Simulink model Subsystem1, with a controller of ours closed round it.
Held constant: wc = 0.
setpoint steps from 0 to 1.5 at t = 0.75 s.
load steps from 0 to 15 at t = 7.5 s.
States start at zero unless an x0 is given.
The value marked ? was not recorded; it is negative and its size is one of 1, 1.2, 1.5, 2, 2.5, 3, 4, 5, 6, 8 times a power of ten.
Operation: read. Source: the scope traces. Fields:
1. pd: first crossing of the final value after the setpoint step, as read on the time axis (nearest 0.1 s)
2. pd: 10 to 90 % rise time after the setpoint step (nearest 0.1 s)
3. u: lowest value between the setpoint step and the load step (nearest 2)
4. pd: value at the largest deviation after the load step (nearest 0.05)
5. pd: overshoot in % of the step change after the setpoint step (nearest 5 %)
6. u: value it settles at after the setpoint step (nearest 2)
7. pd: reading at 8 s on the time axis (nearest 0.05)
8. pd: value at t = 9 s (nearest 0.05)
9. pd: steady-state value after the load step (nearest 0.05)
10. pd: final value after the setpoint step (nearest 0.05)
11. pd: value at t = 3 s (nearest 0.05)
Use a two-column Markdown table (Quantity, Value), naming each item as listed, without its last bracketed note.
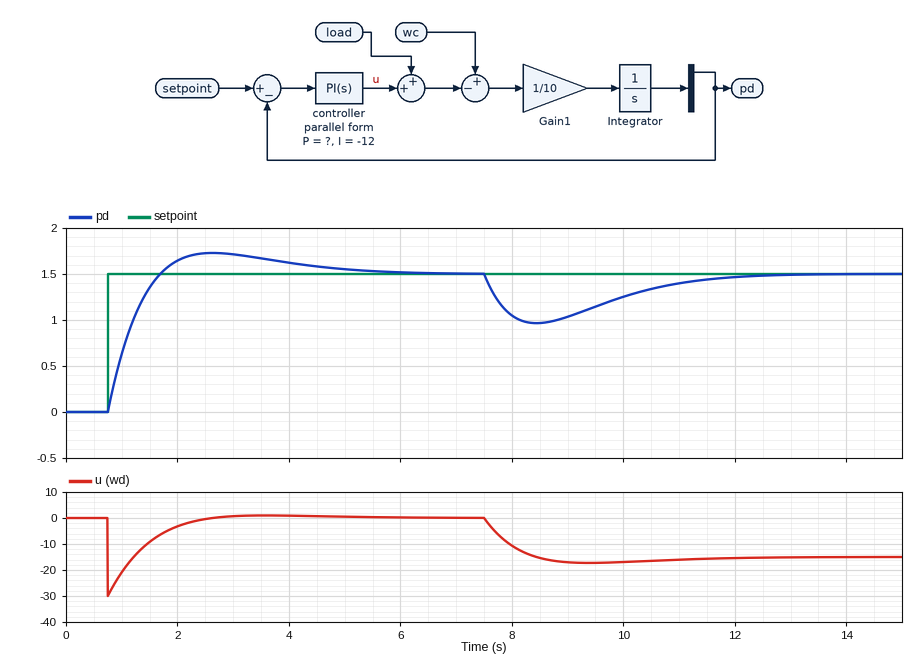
| Quantity | Value |
|---|---|
| pd: first crossing of the final value after the setpoint step, as read on the time axis | 1.7 s |
| pd: 10 to 90 % rise time after the setpoint step | 0.7 s |
| u: lowest value between the setpoint step and the load step | -30 |
| pd: value at the largest deviation after the load step | 0.95 |
| pd: overshoot in % of the step change after the setpoint step | 15 % |
| u: value it settles at after the setpoint step | 0 |
| pd: reading at 8 s on the time axis | 1.05 |
| pd: value at t = 9 s | 1.05 |
| pd: steady-state value after the load step | 1.50 |
| pd: final value after the setpoint step | 1.50 |
| pd: value at t = 3 s | 1.70 |
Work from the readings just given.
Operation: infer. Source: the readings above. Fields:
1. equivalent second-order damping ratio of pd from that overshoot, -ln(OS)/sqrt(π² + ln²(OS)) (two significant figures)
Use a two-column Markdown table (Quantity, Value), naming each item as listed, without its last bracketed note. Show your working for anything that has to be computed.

| Quantity | Value |
|---|---|
| equivalent second-order damping ratio of pd from that overshoot, -ln(OS)/sqrt(π² + ln²(OS)) | ln(0.15) = -1.897; 1.897 / sqrt(9.870 + 3.599) = 0.52 |
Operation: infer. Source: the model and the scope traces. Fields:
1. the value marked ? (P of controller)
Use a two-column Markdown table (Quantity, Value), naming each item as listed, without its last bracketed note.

| Quantity | Value |
|---|---|
| the value marked ? | -20 |
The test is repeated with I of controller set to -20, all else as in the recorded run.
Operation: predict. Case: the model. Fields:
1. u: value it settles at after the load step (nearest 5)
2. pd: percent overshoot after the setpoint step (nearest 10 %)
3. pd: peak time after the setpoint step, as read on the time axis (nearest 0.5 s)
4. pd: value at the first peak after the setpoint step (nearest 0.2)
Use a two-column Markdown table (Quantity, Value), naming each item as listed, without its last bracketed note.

| Quantity | Value |
|---|---|
| u: value it settles at after the load step | -15 |
| pd: percent overshoot after the setpoint step | 20 % |
| pd: peak time after the setpoint step, as read on the time axis | 2.5 s |
| pd: value at the first peak after the setpoint step | 1.8 |
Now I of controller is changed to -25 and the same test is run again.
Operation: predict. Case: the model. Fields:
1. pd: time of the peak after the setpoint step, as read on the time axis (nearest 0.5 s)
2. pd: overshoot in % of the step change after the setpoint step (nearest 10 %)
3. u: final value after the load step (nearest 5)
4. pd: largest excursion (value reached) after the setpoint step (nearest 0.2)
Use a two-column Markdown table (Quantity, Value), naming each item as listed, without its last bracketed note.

| Quantity | Value |
|---|---|
| pd: time of the peak after the setpoint step, as read on the time axis | 2.0 s |
| pd: overshoot in % of the step change after the setpoint step | 20 % |
| u: final value after the load step | -15 |
| pd: largest excursion (value reached) after the setpoint step | 1.8 |
